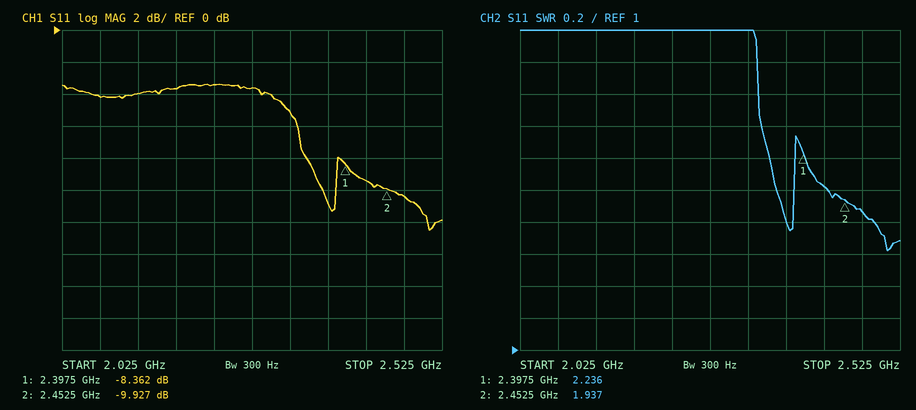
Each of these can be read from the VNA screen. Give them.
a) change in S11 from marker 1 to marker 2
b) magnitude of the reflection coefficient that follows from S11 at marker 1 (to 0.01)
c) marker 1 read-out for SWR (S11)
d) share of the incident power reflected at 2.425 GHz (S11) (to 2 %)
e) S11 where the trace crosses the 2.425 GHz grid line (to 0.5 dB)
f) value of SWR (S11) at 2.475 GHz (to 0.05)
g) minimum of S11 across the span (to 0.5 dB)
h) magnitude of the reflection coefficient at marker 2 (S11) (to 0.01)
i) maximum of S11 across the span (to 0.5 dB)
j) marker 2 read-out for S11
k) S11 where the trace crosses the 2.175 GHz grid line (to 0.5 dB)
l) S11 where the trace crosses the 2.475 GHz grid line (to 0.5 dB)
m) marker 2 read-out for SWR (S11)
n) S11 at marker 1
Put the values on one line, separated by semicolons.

-1.565 dB; 0.38; 2.236; 12 %; -9.5 dB; 1.85; -12.5 dB; 0.32; -3.5 dB; -9.927 dB; -3.5 dB; -10.5 dB; 1.937; -8.362 dB
